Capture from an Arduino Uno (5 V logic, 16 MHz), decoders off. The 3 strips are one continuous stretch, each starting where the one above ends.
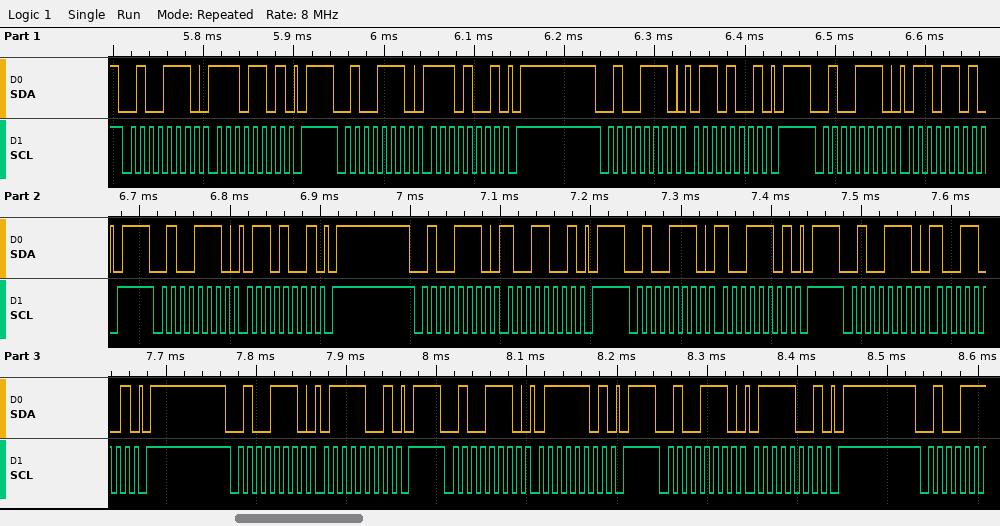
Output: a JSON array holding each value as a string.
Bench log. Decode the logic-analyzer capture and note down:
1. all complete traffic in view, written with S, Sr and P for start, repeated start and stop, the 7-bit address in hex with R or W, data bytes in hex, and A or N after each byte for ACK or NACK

["S 27W A ED A P S 27W A E9 A P S 27W A 69 A P S 27W A 6D A P S 27W A 69 A P S 27W A 99 A P S 27W A 9D A P S 27W A 99 A P S 27W A 79 A P S 27W A 7D A P S 27W A 79 A P"]
